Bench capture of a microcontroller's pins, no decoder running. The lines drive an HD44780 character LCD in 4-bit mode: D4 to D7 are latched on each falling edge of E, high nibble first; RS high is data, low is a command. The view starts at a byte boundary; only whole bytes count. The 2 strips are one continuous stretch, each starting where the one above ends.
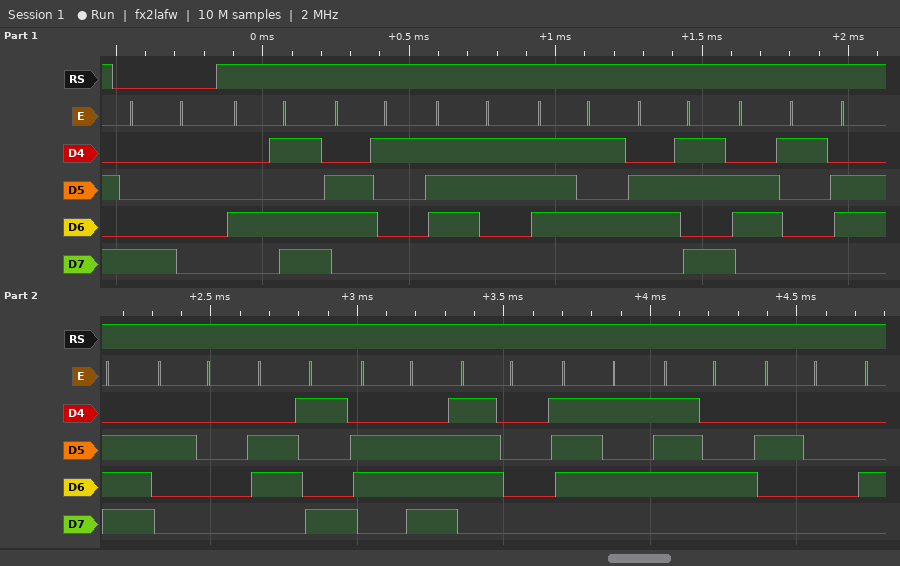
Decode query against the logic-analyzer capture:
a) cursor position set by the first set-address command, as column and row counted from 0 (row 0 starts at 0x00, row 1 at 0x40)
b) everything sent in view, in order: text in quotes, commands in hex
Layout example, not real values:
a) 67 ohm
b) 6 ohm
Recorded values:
a) column 0, row 0
b) 0x80 "Masukan input "
